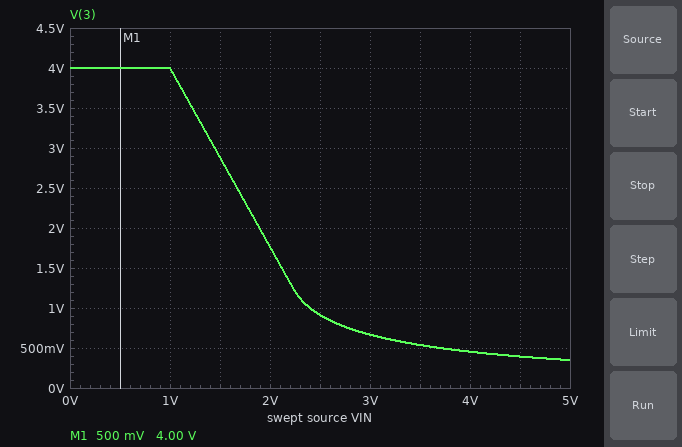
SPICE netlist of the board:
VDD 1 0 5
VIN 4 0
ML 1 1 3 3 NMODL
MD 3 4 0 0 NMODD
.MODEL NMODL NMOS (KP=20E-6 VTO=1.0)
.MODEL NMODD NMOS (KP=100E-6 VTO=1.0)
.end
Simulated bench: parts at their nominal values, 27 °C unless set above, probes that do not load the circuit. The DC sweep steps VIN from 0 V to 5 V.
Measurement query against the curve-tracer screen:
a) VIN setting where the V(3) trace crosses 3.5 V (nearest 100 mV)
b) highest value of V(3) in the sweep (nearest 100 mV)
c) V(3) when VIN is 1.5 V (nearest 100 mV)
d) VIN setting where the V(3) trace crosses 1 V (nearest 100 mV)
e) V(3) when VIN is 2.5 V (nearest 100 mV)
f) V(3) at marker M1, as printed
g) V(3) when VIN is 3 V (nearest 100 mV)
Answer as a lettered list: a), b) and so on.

a) 1.2 V
b) 4.0 V
c) 2.9 V
d) 2.4 V
e) 900 mV
f) 4.00 V
g) 700 mV
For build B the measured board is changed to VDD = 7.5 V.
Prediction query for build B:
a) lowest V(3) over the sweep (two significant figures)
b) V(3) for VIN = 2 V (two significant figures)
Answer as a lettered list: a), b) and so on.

a) 890 mV
b) 4.3 V
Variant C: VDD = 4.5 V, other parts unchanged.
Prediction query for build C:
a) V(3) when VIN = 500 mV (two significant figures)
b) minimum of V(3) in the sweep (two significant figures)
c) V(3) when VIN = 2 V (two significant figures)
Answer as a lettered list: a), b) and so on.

a) 3.5 V
b) 270 mV
c) 1.3 V
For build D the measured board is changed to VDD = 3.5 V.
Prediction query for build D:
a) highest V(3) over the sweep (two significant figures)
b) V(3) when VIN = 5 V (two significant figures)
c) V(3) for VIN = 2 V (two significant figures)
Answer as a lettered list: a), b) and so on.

a) 2.5 V
b) 140 mV
c) 530 mV
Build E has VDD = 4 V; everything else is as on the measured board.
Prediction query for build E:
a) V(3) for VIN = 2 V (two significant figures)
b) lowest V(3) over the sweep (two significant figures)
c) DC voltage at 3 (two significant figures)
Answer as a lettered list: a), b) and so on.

a) 810 mV
b) 200 mV
c) 3.0 V
